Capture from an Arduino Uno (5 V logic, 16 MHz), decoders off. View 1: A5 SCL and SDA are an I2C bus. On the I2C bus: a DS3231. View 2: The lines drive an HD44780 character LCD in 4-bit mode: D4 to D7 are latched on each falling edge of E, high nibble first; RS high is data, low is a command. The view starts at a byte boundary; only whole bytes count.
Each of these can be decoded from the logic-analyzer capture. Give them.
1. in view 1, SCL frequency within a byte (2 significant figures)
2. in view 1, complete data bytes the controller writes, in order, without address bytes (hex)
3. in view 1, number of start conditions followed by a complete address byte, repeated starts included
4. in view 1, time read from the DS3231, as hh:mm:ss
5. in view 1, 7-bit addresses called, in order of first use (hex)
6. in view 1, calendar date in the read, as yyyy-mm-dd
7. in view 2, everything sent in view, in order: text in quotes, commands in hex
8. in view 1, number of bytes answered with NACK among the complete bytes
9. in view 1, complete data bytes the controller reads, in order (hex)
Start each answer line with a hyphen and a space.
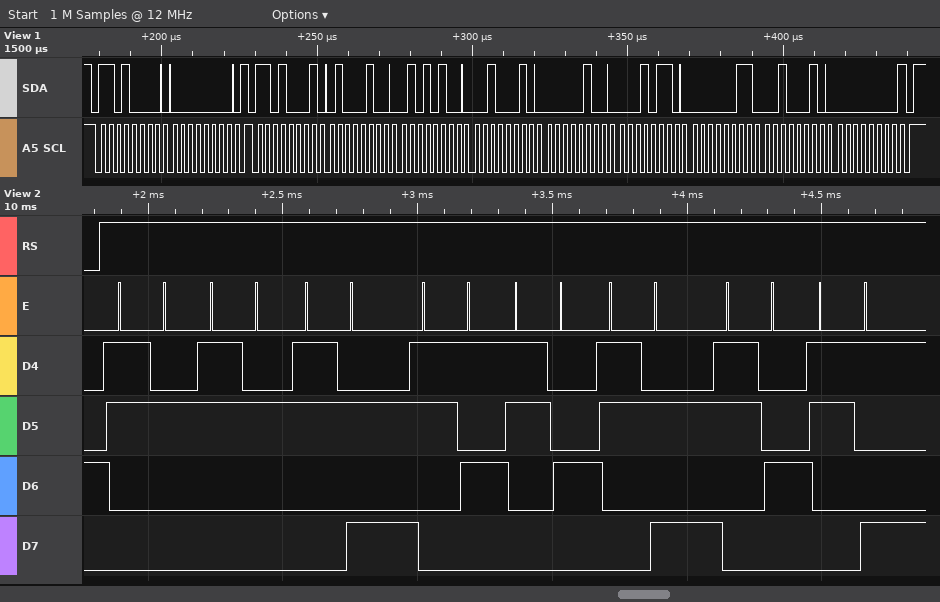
- 400 kHz
- 00
- 2
- 22:54:44
- 0x68
- 2022-03-16
- "22:54:49"
- 1
- 44 54 22 04 16 03 22 00
